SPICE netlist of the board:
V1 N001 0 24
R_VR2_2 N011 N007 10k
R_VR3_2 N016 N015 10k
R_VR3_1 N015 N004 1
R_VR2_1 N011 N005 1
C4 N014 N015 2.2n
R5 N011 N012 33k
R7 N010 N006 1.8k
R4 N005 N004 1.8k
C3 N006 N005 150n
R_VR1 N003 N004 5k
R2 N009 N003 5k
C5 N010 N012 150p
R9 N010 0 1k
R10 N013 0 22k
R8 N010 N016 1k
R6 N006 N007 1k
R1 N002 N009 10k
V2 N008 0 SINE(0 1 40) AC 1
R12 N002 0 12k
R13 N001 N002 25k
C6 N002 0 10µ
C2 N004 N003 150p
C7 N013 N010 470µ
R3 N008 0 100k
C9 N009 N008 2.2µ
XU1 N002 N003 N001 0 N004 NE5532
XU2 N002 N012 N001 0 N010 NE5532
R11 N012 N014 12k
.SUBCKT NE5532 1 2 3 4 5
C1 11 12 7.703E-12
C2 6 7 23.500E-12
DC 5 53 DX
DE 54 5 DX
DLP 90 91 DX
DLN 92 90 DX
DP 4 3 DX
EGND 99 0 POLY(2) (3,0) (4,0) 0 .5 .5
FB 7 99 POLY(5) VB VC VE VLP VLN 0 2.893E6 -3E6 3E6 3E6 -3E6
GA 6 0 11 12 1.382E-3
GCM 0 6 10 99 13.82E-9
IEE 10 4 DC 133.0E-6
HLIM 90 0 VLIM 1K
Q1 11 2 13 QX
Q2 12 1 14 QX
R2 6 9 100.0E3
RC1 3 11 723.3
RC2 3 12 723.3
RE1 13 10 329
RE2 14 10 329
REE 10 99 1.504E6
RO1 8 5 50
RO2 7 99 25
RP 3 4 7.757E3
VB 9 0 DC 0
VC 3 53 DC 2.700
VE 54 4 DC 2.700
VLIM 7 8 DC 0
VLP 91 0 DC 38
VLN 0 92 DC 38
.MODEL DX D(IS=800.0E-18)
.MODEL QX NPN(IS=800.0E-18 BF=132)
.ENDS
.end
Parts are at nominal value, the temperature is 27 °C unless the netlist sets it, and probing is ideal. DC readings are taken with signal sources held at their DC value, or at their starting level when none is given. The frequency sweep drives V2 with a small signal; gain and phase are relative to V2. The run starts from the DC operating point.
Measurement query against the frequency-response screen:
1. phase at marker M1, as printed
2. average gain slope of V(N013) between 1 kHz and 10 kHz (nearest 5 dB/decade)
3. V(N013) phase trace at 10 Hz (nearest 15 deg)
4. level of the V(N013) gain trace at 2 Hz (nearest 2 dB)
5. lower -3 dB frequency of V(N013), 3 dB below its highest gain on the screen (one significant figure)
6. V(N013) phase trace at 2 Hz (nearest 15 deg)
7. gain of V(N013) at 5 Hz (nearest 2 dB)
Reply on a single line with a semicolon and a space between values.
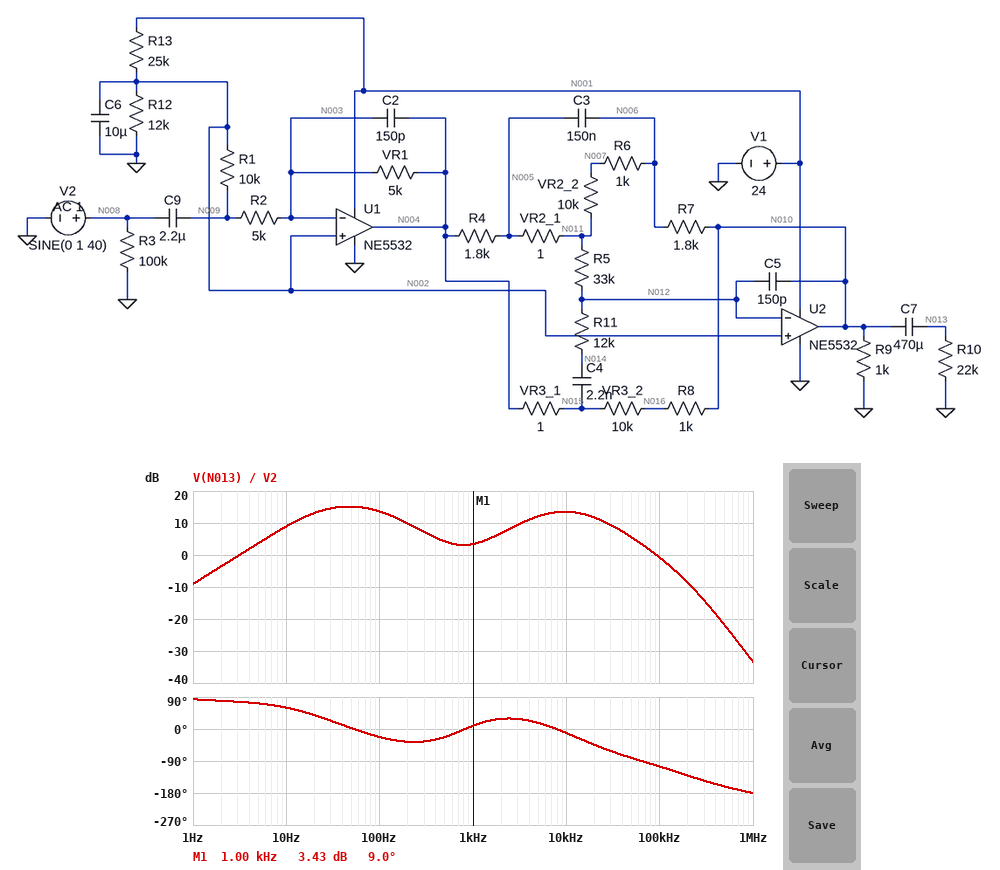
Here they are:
9.0 deg; 10 dB/decade; 60 deg; -4 dB; 20 Hz; 75 deg; 4 dB
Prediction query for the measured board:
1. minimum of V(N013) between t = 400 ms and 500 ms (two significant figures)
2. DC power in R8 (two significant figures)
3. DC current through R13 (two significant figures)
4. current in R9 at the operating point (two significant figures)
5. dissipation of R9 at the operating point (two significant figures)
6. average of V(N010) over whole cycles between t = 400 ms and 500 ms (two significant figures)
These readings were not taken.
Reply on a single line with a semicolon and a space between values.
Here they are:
-5.7 V; 110 nW; 650 µA; 7.9 mA; 62 mW; 7.9 V
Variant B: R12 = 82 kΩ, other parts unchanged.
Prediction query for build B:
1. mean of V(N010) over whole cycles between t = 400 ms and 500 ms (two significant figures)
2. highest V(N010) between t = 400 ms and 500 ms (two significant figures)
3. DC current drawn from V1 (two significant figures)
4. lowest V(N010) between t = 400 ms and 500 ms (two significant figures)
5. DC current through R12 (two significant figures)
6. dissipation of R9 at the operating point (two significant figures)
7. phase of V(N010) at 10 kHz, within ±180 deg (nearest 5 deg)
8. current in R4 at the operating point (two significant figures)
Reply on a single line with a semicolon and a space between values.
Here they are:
18 V; 22 V; 6.7 mA; 13 V; 220 µA; 340 mW; -10 deg; 8.0 µA
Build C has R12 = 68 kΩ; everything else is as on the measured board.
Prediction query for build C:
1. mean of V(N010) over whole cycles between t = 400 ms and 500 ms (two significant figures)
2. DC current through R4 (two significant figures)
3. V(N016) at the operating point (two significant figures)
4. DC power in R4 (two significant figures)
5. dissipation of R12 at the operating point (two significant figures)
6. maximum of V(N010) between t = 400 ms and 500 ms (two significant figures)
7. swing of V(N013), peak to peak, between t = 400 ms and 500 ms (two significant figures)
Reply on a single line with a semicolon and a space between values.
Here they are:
17 V; 8.0 µA; 18 V; 110 nW; 4.5 mW; 22 V; 10 V
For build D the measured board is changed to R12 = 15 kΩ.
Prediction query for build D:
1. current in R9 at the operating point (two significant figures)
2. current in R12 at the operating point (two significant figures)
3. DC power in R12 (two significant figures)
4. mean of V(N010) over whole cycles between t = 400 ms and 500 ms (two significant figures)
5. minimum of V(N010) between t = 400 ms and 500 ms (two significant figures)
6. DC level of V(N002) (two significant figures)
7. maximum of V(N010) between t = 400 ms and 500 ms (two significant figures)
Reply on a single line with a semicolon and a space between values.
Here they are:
9.1 mA; 600 µA; 5.4 mW; 9.1 V; 3.4 V; 9.0 V; 15 V
